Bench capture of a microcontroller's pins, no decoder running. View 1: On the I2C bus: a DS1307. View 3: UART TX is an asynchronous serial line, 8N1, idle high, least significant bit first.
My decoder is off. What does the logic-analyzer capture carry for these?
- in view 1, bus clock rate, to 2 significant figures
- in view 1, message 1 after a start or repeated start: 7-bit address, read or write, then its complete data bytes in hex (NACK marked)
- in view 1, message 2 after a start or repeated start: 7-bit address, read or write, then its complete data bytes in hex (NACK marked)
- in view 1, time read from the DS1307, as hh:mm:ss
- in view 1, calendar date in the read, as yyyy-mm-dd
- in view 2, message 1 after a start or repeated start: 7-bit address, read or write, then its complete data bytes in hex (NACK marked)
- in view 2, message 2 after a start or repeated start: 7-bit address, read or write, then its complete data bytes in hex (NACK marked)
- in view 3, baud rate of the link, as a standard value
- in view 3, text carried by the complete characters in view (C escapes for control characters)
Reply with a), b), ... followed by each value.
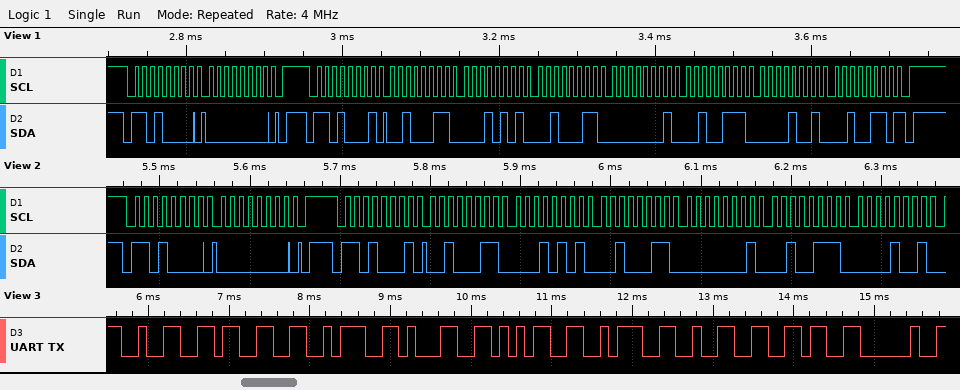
a) 100 kHz
b) 0x68 write: 00
c) 0x68 read: 23 15 23 01 27 09 26 NACK
d) 23:15:23
e) 2026-09-27
f) 0x68 write: 00
g) 0x68 read: 23 15 23 01 27 09
h) 9600 baud
i) "23:15:26 "
